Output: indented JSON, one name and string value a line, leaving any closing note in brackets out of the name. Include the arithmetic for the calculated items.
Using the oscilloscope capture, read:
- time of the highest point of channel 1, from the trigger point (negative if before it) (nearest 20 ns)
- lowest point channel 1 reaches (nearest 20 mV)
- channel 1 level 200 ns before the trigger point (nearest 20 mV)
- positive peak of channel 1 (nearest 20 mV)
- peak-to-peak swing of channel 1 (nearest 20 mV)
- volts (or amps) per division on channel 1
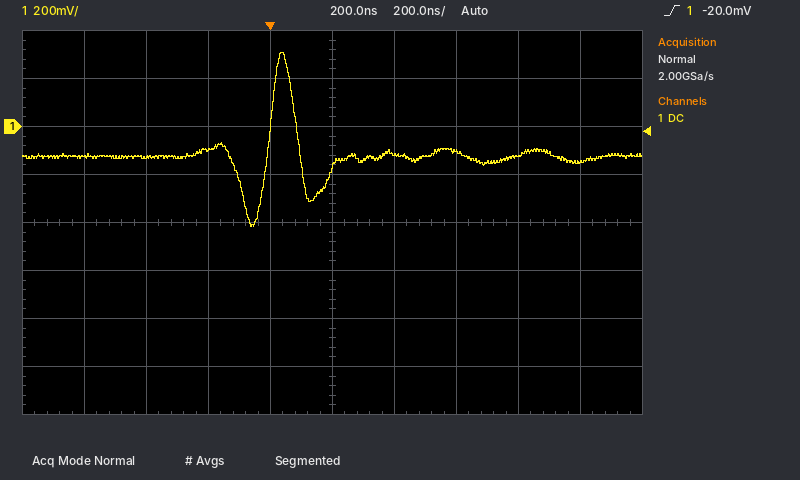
{
  "time of the highest point of channel 1, from the trigger point (negative if before it)": "+40 ns",
  "lowest point channel 1 reaches": "-420 mV",
  "channel 1 level 200 ns before the trigger point": "-100 mV",
  "positive peak of channel 1": "300 mV",
  "peak-to-peak swing of channel 1": "300 mV − (-420 mV) = 720 mV",
  "volts (or amps) per division on channel 1": "200 mV"
}
